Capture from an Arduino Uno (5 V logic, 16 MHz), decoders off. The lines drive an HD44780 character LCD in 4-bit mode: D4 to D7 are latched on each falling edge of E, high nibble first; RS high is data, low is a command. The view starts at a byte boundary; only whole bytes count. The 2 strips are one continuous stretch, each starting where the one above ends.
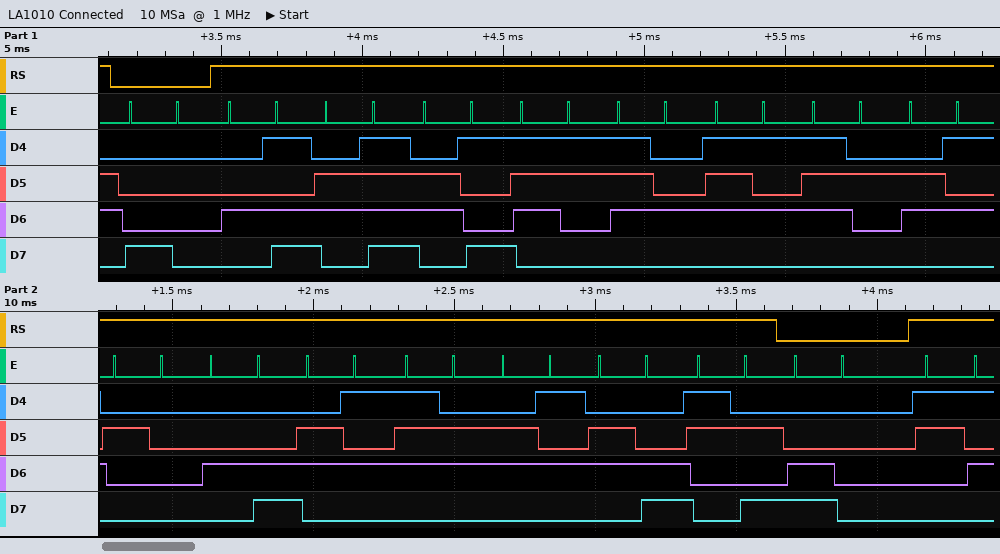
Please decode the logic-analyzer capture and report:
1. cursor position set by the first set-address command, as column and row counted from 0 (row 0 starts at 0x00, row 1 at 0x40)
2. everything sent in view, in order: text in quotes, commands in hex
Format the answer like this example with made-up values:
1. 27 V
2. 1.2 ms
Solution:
1. column 0, row 0
2. 0x80 "Moisture Level:" 0xC0 "5"
